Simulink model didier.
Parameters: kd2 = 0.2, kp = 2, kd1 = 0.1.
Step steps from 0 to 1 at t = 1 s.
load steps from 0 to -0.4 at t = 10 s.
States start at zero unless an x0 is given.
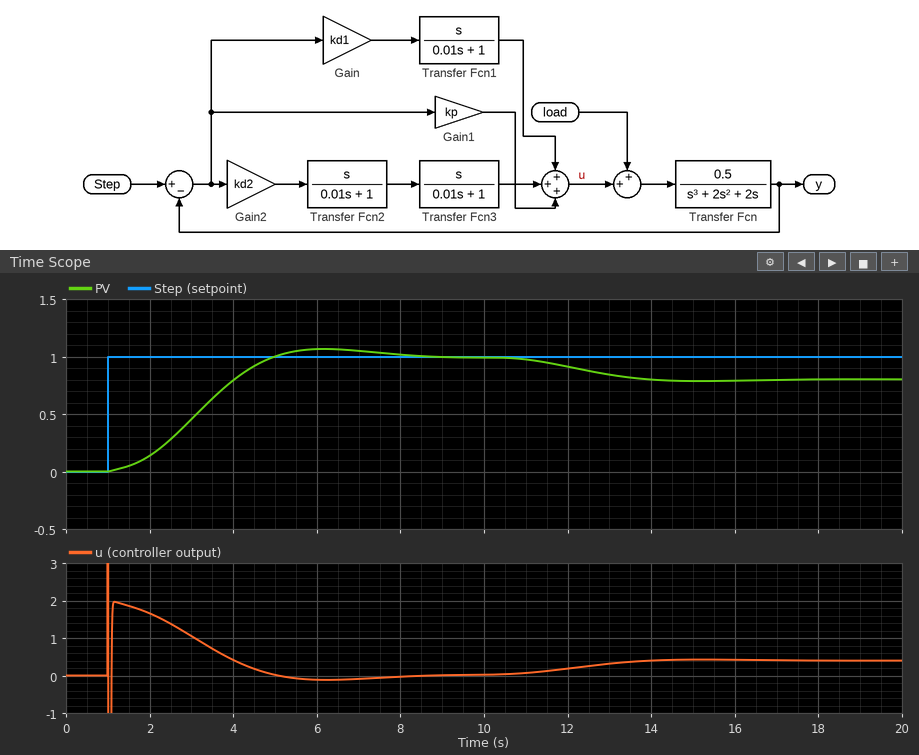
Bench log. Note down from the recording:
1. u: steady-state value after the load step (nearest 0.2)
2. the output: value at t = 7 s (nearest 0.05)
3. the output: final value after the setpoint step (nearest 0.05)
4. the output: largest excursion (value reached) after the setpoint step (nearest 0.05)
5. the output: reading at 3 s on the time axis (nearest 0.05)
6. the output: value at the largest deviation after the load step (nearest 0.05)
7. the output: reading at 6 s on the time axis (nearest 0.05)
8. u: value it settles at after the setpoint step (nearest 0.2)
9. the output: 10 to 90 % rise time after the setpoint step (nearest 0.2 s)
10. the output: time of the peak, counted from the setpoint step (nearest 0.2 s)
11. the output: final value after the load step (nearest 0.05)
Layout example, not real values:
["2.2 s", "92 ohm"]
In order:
["0.4", "1.05", "1.00", "1.05", "0.45", "0.80", "1.05", "0.0", "2.6 s", "5.2 s", "0.80"]
